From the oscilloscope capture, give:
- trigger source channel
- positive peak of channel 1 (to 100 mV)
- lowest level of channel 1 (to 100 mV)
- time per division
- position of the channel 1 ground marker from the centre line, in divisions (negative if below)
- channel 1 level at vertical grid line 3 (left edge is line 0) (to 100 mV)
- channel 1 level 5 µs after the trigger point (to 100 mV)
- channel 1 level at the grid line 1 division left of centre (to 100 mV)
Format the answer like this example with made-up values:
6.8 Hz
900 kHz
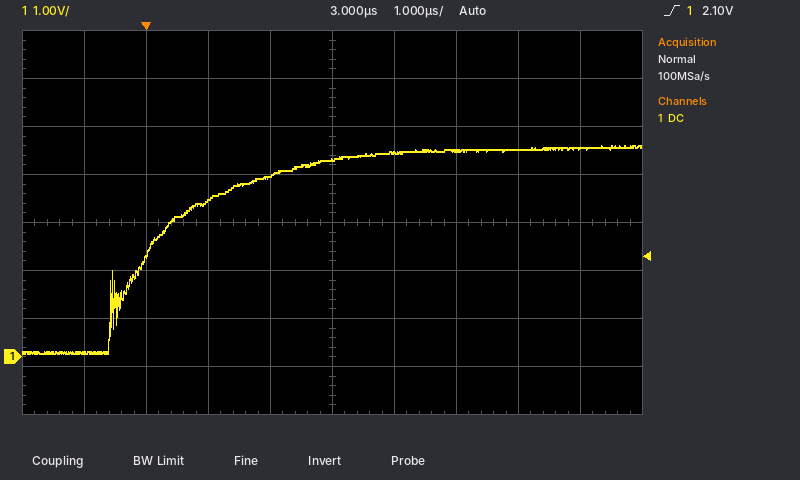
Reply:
channel 1
4.4 V
100 mV
1 µs
-2.8 div
3.3 V
4.3 V
3.8 V
